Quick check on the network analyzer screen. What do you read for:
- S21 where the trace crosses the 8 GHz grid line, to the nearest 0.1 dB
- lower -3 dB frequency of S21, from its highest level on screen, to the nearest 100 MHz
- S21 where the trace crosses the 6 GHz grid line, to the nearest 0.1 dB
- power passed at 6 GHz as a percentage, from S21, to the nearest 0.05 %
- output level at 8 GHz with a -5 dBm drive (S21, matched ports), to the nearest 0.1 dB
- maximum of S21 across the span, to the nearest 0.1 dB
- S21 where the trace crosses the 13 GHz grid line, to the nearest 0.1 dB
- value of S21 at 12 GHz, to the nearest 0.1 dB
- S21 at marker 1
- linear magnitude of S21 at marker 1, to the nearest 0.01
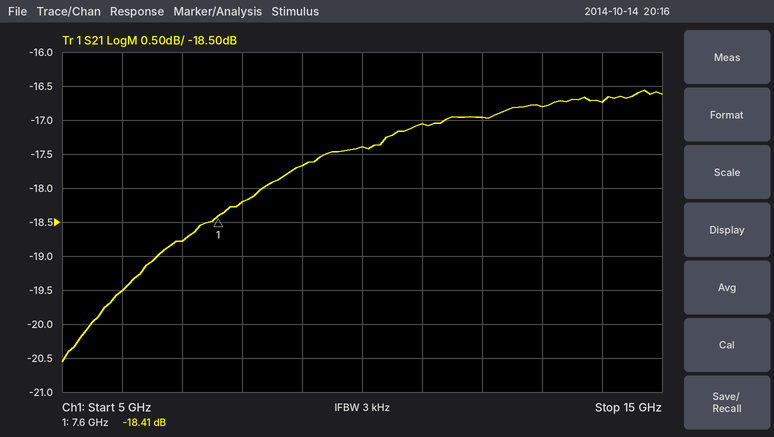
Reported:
-18.2 dB
5.9 GHz
-19.5 dB
1.10 %
-23.2 dBm
-16.6 dB
-16.8 dB
-17.0 dB
-18.41 dB
0.12
